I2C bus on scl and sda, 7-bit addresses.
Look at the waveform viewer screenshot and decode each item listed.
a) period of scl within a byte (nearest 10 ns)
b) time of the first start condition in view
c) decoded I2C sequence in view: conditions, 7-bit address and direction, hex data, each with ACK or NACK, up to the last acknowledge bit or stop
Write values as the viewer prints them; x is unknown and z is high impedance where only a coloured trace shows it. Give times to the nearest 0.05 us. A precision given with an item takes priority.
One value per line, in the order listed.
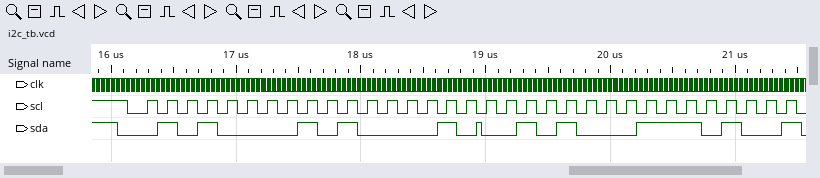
160 ns
16.05 us
start, address 28 write NACK, 42 ACK, 51 NACK
